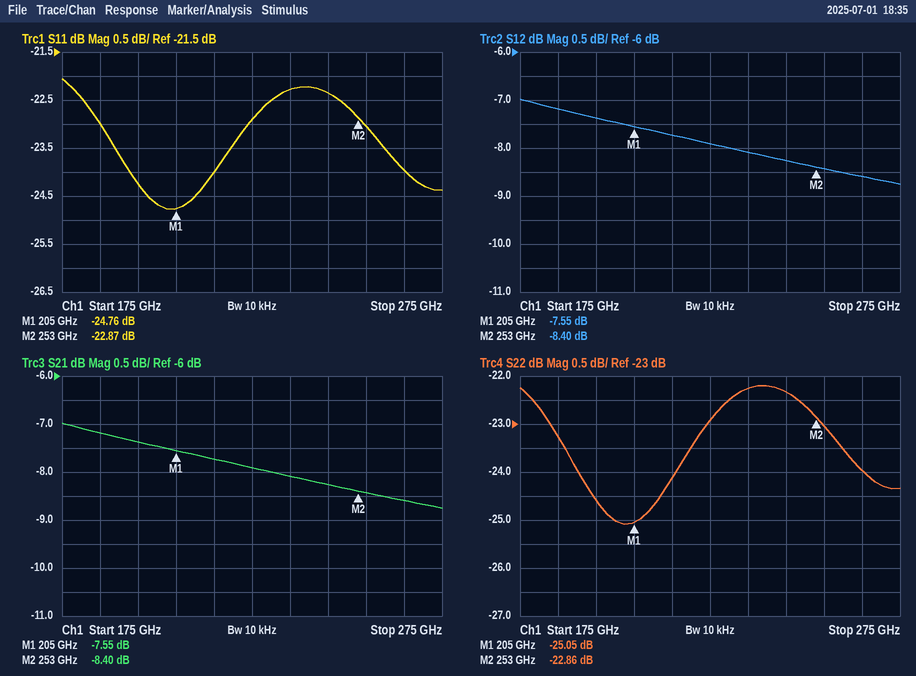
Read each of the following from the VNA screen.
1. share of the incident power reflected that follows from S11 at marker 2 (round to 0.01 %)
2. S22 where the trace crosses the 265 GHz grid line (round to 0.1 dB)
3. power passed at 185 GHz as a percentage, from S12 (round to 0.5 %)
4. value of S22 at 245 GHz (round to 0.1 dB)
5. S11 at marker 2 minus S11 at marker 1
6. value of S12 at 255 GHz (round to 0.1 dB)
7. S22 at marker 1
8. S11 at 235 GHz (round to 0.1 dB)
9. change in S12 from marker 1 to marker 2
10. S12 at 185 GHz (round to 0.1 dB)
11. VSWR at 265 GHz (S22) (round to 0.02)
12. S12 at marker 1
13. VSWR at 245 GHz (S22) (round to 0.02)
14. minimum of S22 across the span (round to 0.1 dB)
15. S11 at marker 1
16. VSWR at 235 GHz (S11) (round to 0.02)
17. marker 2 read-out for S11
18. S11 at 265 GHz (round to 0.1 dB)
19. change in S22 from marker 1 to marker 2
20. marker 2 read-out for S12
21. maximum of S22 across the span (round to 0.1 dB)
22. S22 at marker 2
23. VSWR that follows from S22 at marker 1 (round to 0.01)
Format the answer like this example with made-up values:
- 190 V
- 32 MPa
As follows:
- 0.52 %
- -24.0 dB
- 19.0 %
- -22.3 dB
- 1.89 dB
- -8.4 dB
- -25.05 dB
- -22.3 dB
- -0.85 dB
- -7.2 dB
- 1.14
- -7.55 dB
- 1.16
- -25.1 dB
- -24.76 dB
- 1.16
- -22.87 dB
- -24.0 dB
- 2.19 dB
- -8.40 dB
- -22.2 dB
- -22.86 dB
- 1.12
